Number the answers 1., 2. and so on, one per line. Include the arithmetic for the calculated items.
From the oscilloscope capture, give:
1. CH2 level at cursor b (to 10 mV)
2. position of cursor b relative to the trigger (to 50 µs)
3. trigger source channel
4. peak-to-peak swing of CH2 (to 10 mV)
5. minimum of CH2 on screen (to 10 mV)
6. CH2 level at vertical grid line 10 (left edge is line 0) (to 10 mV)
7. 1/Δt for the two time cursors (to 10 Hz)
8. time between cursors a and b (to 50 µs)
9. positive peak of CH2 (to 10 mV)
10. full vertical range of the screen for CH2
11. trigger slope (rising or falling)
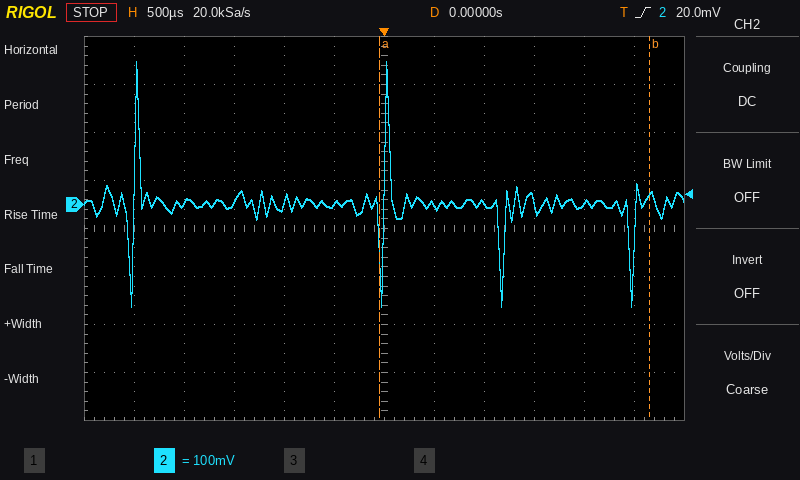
1. 20 mV
2. +2.65 ms
3. CH2
4. 300 mV − (-210 mV) = 510 mV
5. -210 mV
6. 0 mV
7. 1 / 2.70 ms ≈ 370 Hz
8. 2.70 ms
9. 300 mV
10. 800 mV
11. rising
